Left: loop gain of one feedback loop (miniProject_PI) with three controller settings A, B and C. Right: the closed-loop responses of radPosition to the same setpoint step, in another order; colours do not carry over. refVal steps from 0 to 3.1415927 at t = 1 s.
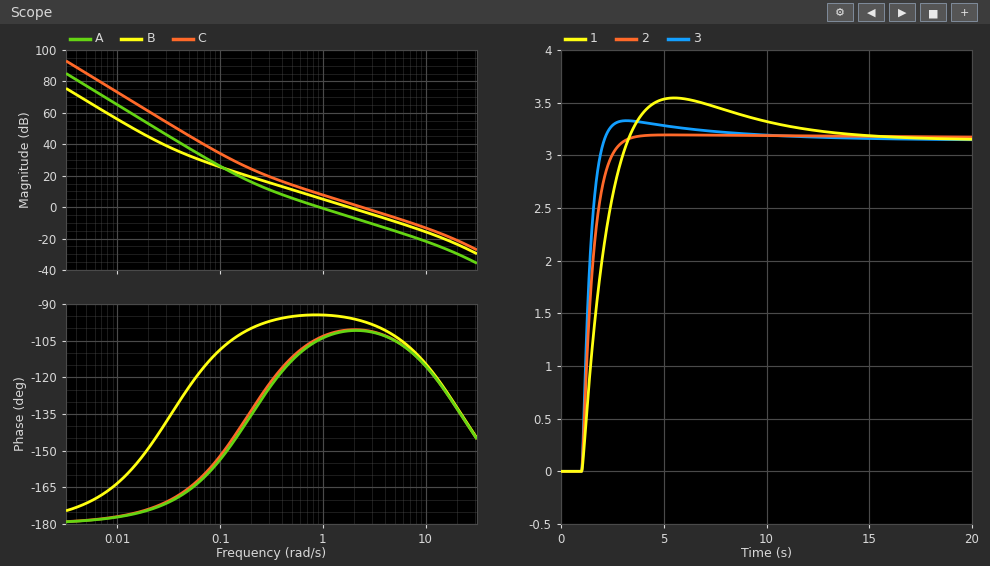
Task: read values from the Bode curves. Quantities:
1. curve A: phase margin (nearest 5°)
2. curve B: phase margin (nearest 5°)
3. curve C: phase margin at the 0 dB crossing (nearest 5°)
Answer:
75°
85°
80°
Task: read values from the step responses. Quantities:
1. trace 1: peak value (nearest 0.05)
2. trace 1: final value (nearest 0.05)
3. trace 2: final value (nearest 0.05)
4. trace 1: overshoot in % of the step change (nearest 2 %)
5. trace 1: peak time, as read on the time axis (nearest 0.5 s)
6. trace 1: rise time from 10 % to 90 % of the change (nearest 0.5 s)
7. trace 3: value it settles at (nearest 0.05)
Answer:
3.55
3.15
3.15
12 %
5.5 s
1.5 s
3.15
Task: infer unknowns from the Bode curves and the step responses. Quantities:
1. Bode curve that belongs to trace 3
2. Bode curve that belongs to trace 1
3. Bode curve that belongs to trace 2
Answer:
C
A
B
